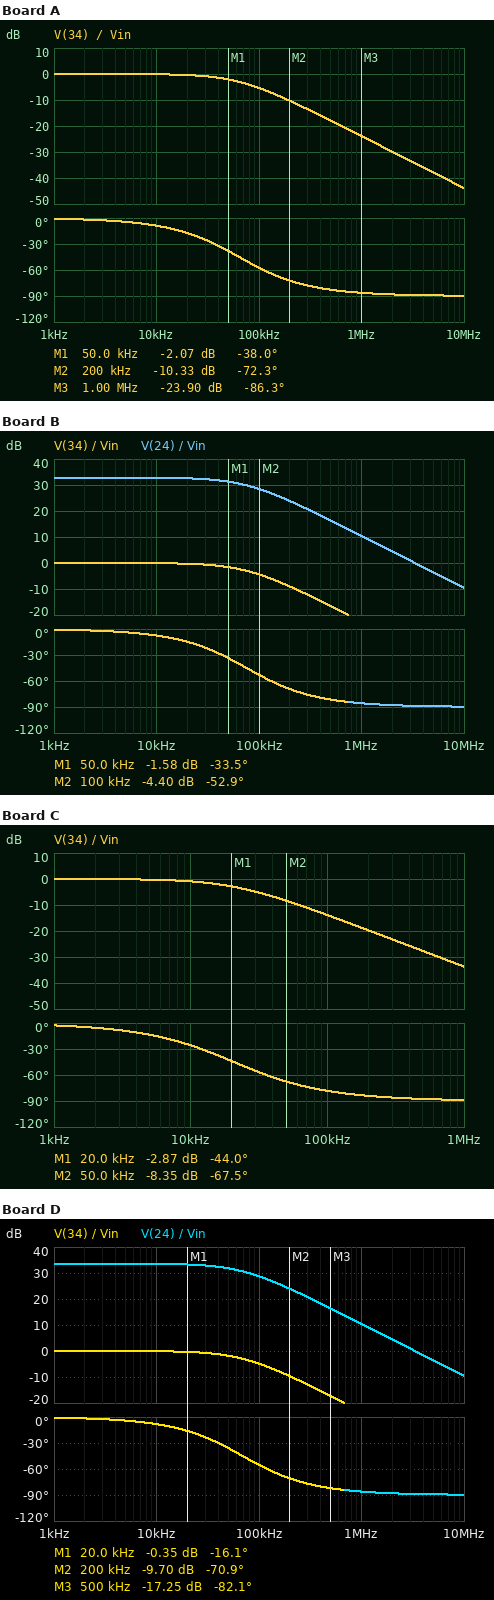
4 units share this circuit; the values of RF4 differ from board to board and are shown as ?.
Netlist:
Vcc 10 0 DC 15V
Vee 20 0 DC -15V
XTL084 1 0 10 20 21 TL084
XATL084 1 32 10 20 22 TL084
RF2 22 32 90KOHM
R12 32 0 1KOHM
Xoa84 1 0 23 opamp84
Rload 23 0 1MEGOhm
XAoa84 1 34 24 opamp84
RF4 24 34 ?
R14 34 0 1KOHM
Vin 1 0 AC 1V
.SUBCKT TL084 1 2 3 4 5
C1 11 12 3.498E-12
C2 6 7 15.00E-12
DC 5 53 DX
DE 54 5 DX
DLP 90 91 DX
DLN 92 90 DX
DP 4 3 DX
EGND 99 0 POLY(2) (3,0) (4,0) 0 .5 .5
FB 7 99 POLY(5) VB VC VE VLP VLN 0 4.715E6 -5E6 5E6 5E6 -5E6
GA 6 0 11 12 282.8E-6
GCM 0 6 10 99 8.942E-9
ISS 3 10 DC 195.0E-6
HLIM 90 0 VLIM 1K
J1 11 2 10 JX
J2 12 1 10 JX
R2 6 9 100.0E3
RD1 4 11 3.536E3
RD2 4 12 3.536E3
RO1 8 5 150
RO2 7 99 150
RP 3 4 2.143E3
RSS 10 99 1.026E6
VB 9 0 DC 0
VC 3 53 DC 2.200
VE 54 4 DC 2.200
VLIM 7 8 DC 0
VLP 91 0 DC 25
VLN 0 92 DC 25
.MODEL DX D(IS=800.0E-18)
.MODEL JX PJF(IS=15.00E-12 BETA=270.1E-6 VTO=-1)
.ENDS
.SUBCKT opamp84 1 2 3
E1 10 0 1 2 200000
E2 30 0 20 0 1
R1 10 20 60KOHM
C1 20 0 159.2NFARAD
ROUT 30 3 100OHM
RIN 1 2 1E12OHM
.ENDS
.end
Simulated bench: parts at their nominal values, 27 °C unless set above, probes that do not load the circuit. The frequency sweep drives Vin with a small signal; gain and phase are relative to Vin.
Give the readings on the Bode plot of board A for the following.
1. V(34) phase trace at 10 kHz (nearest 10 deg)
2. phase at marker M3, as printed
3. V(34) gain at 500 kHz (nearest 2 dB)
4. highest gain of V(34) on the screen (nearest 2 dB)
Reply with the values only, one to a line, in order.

-10 deg
-86.3 deg
-18 dB
0 dB
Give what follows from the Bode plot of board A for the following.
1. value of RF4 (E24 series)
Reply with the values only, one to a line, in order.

51 kΩ
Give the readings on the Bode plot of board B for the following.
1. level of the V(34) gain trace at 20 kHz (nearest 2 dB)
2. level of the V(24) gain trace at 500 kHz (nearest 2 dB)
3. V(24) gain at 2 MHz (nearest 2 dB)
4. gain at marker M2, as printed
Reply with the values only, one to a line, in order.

0 dB
16 dB
4 dB
-4.40 dB
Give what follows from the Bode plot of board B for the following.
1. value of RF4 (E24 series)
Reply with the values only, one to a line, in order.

43 kΩ
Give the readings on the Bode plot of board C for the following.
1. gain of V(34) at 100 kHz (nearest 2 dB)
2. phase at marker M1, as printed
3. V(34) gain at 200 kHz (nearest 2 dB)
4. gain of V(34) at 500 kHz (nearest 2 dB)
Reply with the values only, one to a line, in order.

-14 dB
-44.0 deg
-20 dB
-28 dB
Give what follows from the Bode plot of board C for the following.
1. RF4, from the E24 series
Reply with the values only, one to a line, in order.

160 kΩ
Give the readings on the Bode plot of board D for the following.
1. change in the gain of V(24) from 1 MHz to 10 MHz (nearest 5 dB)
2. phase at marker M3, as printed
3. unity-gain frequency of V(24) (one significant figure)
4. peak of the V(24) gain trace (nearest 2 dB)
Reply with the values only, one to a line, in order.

-20 dB
-82.1 deg
3 MHz
34 dB
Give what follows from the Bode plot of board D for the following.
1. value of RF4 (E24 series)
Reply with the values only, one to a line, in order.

47 kΩ
